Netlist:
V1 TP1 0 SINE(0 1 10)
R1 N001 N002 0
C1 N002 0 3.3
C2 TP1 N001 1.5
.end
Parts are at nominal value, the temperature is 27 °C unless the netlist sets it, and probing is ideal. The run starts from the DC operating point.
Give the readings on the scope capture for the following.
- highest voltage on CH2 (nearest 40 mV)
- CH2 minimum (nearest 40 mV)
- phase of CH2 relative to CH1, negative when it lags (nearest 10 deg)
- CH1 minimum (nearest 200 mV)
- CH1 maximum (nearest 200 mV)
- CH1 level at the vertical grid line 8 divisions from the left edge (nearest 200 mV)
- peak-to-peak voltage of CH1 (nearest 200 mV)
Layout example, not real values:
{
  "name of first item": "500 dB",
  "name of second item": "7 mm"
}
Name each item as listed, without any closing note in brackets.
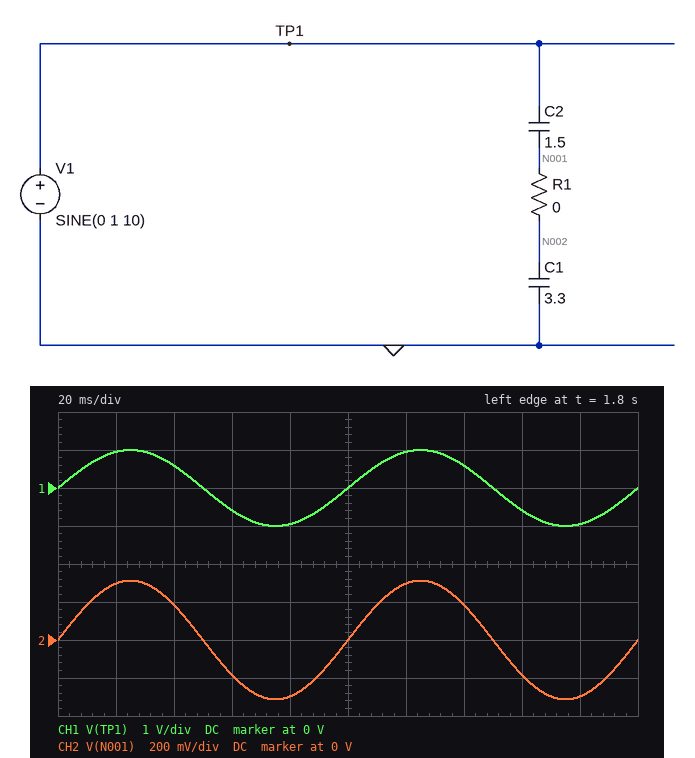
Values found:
{
  "highest voltage on CH2": "320 mV",
  "CH2 minimum": "-320 mV",
  "phase of CH2 relative to CH1, negative when it lags": "0 deg",
  "CH1 minimum": "-1.0 V",
  "CH1 maximum": "1.0 V",
  "CH1 level at the vertical grid line 8 divisions from the left edge": "-600 mV",
  "peak-to-peak voltage of CH1": "2.0 V"
}
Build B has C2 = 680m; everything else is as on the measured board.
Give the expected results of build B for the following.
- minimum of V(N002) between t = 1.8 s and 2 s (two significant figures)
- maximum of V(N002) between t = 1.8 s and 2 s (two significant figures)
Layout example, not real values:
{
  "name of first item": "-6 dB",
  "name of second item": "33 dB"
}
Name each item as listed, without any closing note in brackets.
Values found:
{
  "minimum of V(N002) between t = 1.8 s and 2 s": "-170 mV",
  "maximum of V(N002) between t = 1.8 s and 2 s": "170 mV"
}
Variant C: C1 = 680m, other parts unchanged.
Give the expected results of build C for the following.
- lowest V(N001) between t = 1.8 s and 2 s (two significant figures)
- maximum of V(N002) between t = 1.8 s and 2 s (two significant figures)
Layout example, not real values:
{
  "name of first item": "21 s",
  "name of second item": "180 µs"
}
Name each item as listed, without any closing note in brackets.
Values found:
{
  "lowest V(N001) between t = 1.8 s and 2 s": "-690 mV",
  "maximum of V(N002) between t = 1.8 s and 2 s": "690 mV"
}
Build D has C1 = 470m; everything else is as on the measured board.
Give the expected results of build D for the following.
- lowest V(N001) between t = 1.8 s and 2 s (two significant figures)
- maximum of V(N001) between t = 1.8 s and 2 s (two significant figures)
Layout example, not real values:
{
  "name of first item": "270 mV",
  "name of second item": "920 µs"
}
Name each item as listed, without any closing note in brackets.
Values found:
{
  "lowest V(N001) between t = 1.8 s and 2 s": "-760 mV",
  "maximum of V(N001) between t = 1.8 s and 2 s": "760 mV"
}
